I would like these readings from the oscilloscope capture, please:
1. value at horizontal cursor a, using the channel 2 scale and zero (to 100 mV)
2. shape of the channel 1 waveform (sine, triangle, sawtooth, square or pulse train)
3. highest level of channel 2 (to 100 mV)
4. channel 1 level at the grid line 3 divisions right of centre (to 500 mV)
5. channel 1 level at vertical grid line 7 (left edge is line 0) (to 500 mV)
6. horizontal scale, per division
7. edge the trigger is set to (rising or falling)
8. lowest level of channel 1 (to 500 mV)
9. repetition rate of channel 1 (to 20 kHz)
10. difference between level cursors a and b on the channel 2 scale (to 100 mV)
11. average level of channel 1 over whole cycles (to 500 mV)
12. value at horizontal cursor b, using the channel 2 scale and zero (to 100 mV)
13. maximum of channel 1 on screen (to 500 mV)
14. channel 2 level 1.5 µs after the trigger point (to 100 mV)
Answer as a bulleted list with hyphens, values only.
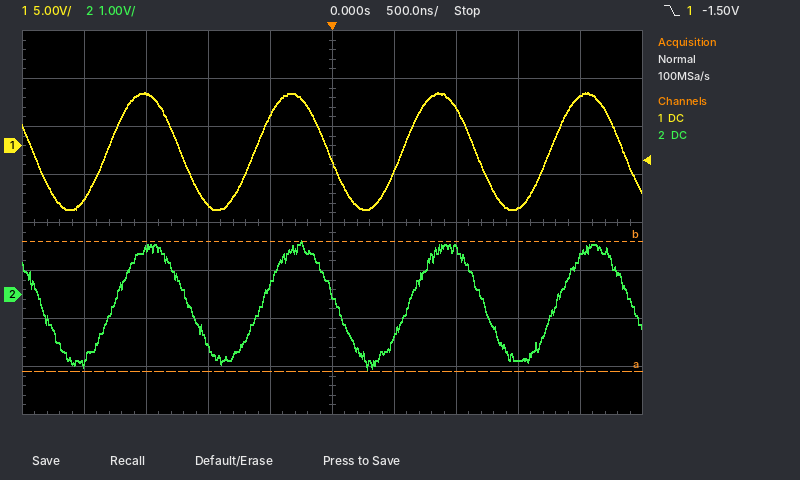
- -1.6 V
- sine
- 1.1 V
- -6.5 V
- 4.0 V
- 500 ns
- falling
- -6.5 V
- 840 kHz
- 2.7 V
- -500 mV
- 1.1 V
- 5.5 V
- -1.4 V
